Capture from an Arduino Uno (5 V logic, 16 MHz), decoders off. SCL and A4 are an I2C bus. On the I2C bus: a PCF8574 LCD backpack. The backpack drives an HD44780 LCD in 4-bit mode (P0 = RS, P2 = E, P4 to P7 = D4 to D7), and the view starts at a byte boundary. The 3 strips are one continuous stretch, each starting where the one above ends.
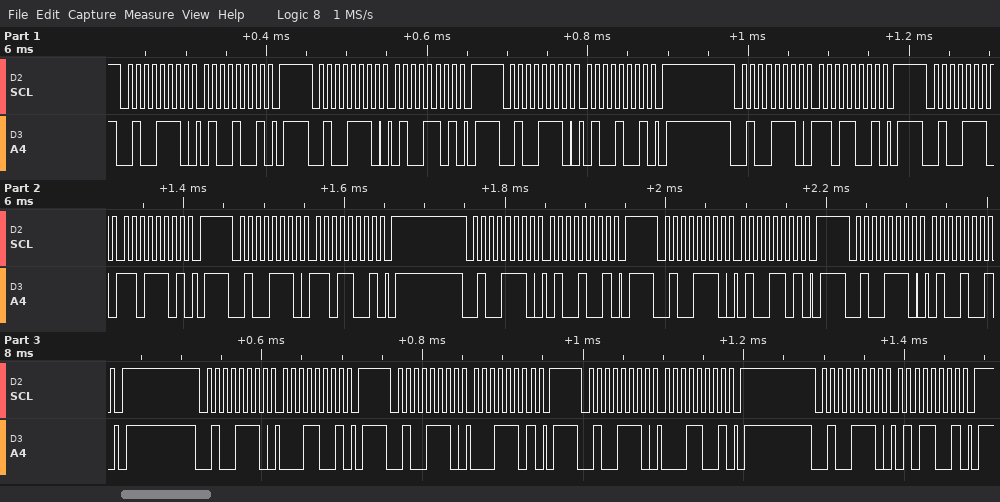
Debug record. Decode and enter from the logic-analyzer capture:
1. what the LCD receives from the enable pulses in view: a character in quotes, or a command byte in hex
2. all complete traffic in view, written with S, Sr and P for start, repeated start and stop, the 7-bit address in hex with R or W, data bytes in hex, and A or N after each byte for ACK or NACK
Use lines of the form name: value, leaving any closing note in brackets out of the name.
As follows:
what the LCD receives from the enable pulses in view: a character in quotes, or a command byte in hex: 'M' 'A'
all complete traffic in view, written with S, Sr and P for start, repeated start and stop, the 7-bit address in hex with R or W, data bytes in hex, and A or N after each byte for ACK or NACK: S 27W A 49 A P S 27W A 4D A P S 27W A 49 A P S 27W A D9 A P S 27W A DD A P S 27W A D9 A P S 27W A 49 A P S 27W A 4D A P S 27W A 49 A P S 27W A 19 A P S 27W A 1D A P S 27W A 19 A P S 27W A 59 A P
